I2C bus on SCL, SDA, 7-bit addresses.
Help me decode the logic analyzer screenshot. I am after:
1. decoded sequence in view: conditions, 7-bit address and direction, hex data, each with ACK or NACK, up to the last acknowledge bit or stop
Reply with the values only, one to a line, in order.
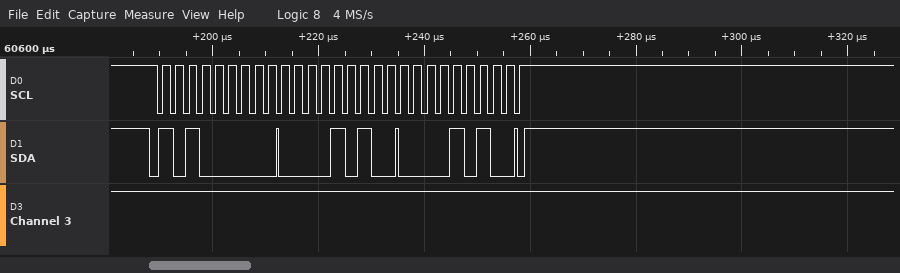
start, address 50 write ACK, 0A ACK, 0A ACK, stop
